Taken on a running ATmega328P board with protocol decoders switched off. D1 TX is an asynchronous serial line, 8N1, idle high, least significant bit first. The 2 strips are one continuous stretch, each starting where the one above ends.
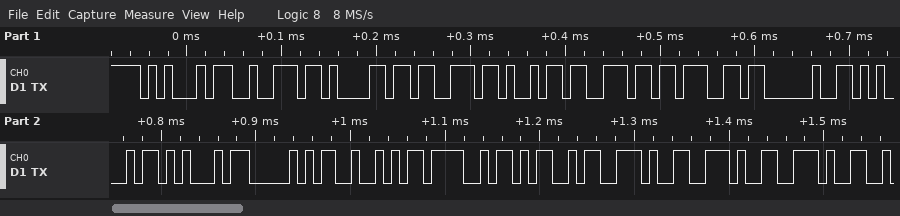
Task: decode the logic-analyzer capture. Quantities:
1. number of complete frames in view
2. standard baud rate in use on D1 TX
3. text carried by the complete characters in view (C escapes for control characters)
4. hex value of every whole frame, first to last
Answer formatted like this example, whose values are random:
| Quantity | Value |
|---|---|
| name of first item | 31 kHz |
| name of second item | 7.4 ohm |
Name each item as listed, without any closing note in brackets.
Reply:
| Quantity | Value |
|---|---|
| number of complete frames in view | 17 |
| standard baud rate in use on D1 TX | 115200 baud |
| text carried by the complete characters in view | "Erasing EEPROM..." |
| hex value of every whole frame, first to last | 0x45 0x72 0x61 0x73 0x69 0x6E 0x67 0x20 0x45 0x45 0x50 0x52 0x4F 0x4D 0x2E 0x2E 0x2E |
